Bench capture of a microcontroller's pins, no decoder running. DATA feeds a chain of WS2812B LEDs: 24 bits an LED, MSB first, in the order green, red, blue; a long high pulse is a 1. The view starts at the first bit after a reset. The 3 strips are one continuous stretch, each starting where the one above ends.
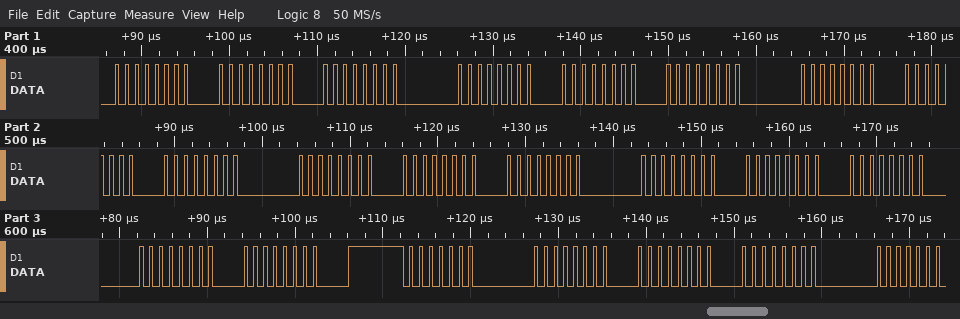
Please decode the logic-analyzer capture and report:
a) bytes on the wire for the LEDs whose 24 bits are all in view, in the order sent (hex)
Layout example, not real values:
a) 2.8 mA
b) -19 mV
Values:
a) 00 00 00 00 00 00 00 00 00 00 00 00 00 00 00 00 00 80 00 00 00
